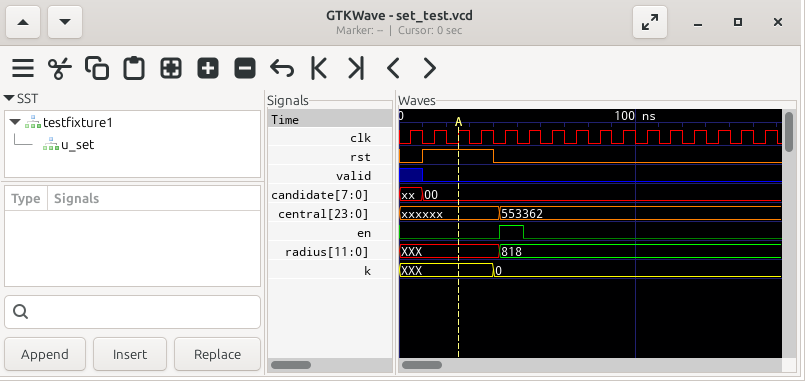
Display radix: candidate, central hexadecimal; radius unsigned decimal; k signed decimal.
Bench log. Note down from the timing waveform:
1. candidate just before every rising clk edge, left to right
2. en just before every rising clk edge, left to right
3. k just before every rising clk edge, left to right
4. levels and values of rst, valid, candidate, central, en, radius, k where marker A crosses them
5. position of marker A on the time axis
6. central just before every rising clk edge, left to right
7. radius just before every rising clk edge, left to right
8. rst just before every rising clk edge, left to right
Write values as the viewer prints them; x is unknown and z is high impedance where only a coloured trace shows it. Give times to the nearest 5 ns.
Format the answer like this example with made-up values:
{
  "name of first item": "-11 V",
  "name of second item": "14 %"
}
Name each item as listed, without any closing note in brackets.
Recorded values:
{
  "candidate just before every rising clk edge, left to right": "xx, 00, 00, 00, 00, 00, 00, 00, 00, 00, 00, 00, 00, 00, 00, 00",
  "en just before every rising clk edge, left to right": "0 0 0 0 1 0 0 0 0 0 0 0 0 0 0 0",
  "k just before every rising clk edge, left to right": "XXX, XXX, XXX, XXX, 0, 0, 0, 0, 0, 0, 0, 0, 0, 0, 0, 0",
  "levels and values of rst, valid, candidate, central, en, radius, k where marker A crosses them": "rst=1, valid=0, candidate=00, central=xxxxxx, en=0, radius=XXX, k=XXX",
  "position of marker A on the time axis": "25 ns",
  "central just before every rising clk edge, left to right": "xxxxxx, xxxxxx, xxxxxx, xxxxxx, 553362, 553362, 553362, 553362, 553362, 553362, 553362, 553362, 553362, 553362, 553362, 553362",
  "radius just before every rising clk edge, left to right": "XXX, XXX, XXX, XXX, 818, 818, 818, 818, 818, 818, 818, 818, 818, 818, 818, 818",
  "rst just before every rising clk edge, left to right": "0 1 1 1 0 0 0 0 0 0 0 0 0 0 0 0"
}
